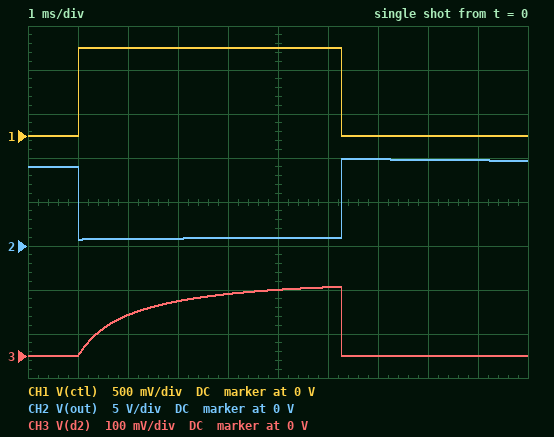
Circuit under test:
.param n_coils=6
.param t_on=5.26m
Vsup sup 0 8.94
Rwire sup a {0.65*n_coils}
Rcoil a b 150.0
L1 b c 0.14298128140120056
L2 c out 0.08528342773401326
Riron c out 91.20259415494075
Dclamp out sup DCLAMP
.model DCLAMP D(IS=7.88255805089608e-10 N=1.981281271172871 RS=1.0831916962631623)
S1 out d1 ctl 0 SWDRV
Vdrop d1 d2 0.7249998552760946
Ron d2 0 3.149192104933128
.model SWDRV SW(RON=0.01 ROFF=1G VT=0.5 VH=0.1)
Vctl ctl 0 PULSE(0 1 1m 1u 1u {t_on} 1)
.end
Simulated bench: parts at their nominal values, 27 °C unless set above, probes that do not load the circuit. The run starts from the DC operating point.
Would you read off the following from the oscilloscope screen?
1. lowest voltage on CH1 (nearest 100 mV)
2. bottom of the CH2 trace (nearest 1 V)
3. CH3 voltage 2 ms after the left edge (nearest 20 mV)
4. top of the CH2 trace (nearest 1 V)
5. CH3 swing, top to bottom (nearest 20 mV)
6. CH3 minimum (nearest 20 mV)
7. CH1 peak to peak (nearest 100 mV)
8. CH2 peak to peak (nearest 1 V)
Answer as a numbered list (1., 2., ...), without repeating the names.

1. 0 V
2. 1 V
3. 100 mV
4. 10 V
5. 160 mV
6. 0 V
7. 1.0 V
8. 9 V
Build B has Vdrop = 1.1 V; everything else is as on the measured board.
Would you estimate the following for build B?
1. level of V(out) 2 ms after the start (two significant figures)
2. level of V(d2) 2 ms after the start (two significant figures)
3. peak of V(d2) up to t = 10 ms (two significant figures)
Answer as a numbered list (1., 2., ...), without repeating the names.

1. 1.2 V
2. 89 mV
3. 150 mV
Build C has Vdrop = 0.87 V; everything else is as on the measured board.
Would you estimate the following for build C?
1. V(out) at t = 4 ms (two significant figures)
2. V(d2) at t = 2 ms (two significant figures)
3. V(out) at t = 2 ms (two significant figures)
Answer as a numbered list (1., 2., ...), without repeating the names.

1. 1.0 V
2. 91 mV
3. 960 mV
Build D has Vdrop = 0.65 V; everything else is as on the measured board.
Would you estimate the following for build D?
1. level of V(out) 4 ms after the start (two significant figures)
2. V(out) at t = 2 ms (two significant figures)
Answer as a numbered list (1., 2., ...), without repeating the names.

1. 790 mV
2. 740 mV
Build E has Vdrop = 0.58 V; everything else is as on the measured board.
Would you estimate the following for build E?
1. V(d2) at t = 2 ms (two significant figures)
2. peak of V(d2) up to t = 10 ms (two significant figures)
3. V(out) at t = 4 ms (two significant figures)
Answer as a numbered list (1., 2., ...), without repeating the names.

1. 95 mV
2. 160 mV
3. 720 mV
